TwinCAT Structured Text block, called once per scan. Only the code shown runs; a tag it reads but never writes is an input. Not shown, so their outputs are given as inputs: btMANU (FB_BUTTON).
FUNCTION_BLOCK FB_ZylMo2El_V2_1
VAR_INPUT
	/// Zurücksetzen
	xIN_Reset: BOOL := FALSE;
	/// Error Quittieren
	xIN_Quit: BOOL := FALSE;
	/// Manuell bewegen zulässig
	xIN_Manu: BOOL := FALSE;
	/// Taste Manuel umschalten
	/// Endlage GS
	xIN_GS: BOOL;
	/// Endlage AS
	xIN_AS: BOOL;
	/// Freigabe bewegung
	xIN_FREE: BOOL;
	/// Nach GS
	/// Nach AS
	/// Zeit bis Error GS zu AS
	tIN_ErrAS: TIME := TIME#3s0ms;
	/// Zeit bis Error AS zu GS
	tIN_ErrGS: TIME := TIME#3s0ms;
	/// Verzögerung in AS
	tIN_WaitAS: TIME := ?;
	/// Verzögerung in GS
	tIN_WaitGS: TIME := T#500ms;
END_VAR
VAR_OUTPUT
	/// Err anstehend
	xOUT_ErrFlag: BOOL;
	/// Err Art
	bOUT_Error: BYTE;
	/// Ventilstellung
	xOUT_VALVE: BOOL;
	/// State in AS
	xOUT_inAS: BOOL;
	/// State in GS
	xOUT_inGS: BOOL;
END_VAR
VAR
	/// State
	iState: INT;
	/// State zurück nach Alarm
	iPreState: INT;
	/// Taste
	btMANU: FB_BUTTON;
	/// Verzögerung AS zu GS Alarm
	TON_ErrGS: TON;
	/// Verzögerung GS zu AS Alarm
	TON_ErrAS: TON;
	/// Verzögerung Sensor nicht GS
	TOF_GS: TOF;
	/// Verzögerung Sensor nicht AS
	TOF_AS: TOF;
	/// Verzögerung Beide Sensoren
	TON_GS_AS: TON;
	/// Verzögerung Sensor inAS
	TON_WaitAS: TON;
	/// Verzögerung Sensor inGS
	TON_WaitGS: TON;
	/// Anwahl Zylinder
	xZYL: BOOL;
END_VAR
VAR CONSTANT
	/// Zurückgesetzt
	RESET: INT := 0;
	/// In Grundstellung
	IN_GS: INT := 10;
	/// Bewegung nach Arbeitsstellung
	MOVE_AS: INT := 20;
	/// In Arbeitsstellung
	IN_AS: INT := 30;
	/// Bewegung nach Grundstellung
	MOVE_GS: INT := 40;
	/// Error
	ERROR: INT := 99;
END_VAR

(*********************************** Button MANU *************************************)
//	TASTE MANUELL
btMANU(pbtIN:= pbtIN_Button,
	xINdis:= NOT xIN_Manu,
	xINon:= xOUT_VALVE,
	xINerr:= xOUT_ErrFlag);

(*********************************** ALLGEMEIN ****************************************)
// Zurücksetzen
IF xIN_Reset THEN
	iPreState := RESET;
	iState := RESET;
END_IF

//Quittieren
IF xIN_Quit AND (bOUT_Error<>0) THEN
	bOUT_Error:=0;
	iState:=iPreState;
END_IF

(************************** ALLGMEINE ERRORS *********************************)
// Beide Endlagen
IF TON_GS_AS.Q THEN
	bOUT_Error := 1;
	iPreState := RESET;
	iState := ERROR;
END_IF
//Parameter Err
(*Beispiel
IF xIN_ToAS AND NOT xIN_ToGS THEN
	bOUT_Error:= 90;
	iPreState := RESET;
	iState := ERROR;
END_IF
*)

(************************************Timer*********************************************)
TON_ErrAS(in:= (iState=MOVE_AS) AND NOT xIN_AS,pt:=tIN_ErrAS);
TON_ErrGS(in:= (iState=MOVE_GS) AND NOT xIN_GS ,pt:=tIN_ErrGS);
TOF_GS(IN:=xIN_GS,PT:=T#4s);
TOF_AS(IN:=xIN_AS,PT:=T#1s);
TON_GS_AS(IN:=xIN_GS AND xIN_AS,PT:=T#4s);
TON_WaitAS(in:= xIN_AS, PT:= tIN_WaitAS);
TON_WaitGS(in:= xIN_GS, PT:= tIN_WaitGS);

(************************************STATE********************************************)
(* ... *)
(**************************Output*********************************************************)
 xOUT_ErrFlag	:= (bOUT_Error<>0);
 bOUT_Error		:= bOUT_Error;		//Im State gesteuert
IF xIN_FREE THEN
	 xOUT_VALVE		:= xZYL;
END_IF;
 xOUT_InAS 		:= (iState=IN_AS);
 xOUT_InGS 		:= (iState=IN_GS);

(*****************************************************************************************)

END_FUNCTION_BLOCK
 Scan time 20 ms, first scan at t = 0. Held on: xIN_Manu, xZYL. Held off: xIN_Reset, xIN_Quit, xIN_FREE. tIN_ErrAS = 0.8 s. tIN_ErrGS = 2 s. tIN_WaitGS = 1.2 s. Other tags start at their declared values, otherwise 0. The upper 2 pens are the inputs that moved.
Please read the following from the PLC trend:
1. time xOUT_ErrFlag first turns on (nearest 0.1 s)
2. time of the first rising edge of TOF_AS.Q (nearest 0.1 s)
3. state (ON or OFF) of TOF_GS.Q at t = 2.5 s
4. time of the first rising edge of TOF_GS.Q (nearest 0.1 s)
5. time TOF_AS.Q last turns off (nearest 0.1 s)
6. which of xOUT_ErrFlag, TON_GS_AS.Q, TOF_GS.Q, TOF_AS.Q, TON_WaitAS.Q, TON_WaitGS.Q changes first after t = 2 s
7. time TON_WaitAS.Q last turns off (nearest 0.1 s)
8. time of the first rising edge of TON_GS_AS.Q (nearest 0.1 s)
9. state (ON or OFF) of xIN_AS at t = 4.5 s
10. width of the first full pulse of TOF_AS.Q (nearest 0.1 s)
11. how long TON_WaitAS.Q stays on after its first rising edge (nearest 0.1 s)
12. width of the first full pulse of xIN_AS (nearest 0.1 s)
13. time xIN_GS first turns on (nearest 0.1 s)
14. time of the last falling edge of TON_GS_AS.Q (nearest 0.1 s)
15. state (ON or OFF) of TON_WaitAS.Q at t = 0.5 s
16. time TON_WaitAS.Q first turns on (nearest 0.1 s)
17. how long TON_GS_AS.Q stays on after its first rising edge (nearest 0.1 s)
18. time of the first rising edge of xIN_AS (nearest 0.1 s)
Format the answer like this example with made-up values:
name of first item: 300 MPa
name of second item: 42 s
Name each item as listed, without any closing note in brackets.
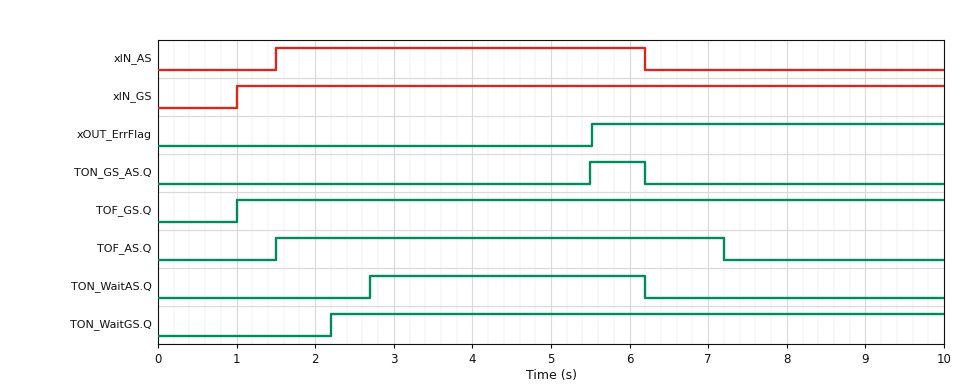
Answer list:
time xOUT_ErrFlag first turns on: 5.5 s
time of the first rising edge of TOF_AS.Q: 1.5 s
state (ON or OFF) of TOF_GS.Q at t = 2.5 s: ON
time of the first rising edge of TOF_GS.Q: 1.0 s
time TOF_AS.Q last turns off: 7.2 s
which of xOUT_ErrFlag, TON_GS_AS.Q, TOF_GS.Q, TOF_AS.Q, TON_WaitAS.Q, TON_WaitGS.Q changes first after t = 2 s: TON_WaitGS.Q
time TON_WaitAS.Q last turns off: 6.2 s
time of the first rising edge of TON_GS_AS.Q: 5.5 s
state (ON or OFF) of xIN_AS at t = 4.5 s: ON
width of the first full pulse of TOF_AS.Q: 5.7 s
how long TON_WaitAS.Q stays on after its first rising edge: 3.5 s
width of the first full pulse of xIN_AS: 4.7 s
time xIN_GS first turns on: 1.0 s
time of the last falling edge of TON_GS_AS.Q: 6.2 s
state (ON or OFF) of TON_WaitAS.Q at t = 0.5 s: OFF
time TON_WaitAS.Q first turns on: 2.7 s
how long TON_GS_AS.Q stays on after its first rising edge: 0.7 s
time of the first rising edge of xIN_AS: 1.5 s
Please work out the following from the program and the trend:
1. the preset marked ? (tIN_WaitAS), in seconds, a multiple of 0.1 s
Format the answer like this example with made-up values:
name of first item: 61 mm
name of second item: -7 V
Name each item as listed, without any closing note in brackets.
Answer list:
the preset marked ? (tIN_WaitAS), in seconds, a multiple of 0.1 s: 1.2 s
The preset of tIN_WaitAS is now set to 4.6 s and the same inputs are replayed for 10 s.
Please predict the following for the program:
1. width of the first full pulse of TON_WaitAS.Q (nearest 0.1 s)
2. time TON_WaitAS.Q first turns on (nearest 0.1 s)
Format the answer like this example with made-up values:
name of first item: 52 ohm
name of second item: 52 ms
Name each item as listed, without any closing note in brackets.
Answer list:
width of the first full pulse of TON_WaitAS.Q: 0.1 s
time TON_WaitAS.Q first turns on: 6.1 s
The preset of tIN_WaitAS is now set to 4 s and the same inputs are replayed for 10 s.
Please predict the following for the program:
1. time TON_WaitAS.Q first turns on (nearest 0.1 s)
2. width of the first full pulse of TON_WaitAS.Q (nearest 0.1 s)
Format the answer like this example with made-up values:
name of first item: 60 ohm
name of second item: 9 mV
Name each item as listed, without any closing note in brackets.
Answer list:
time TON_WaitAS.Q first turns on: 5.5 s
width of the first full pulse of TON_WaitAS.Q: 0.7 s
